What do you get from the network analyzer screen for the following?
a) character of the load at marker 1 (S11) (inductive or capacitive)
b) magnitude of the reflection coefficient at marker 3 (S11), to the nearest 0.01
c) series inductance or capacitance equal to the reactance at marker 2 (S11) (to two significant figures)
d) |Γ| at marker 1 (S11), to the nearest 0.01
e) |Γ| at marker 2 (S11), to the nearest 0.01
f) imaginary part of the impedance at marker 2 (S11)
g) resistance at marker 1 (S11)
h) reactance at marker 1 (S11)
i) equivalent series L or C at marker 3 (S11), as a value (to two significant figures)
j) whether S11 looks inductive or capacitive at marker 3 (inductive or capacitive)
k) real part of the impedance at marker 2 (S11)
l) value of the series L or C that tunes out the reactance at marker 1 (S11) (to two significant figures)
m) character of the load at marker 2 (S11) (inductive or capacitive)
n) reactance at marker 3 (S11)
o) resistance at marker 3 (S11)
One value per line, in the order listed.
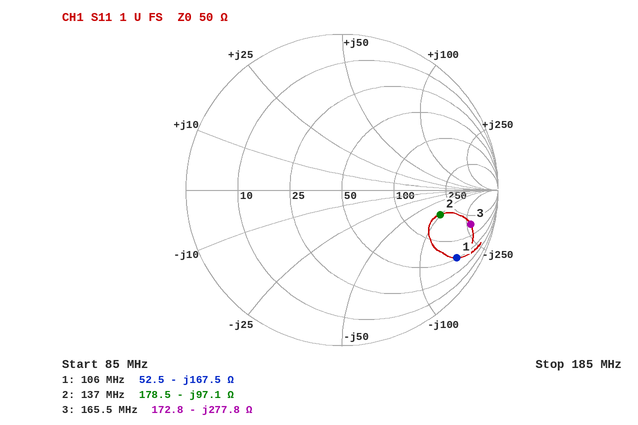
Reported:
capacitive
0.85
12 pF
0.85
0.65
-97.1 Ω
52.5 Ω
-167.5 Ω
3.5 pF
capacitive
178.5 Ω
250 nH
capacitive
-277.8 Ω
172.8 Ω
